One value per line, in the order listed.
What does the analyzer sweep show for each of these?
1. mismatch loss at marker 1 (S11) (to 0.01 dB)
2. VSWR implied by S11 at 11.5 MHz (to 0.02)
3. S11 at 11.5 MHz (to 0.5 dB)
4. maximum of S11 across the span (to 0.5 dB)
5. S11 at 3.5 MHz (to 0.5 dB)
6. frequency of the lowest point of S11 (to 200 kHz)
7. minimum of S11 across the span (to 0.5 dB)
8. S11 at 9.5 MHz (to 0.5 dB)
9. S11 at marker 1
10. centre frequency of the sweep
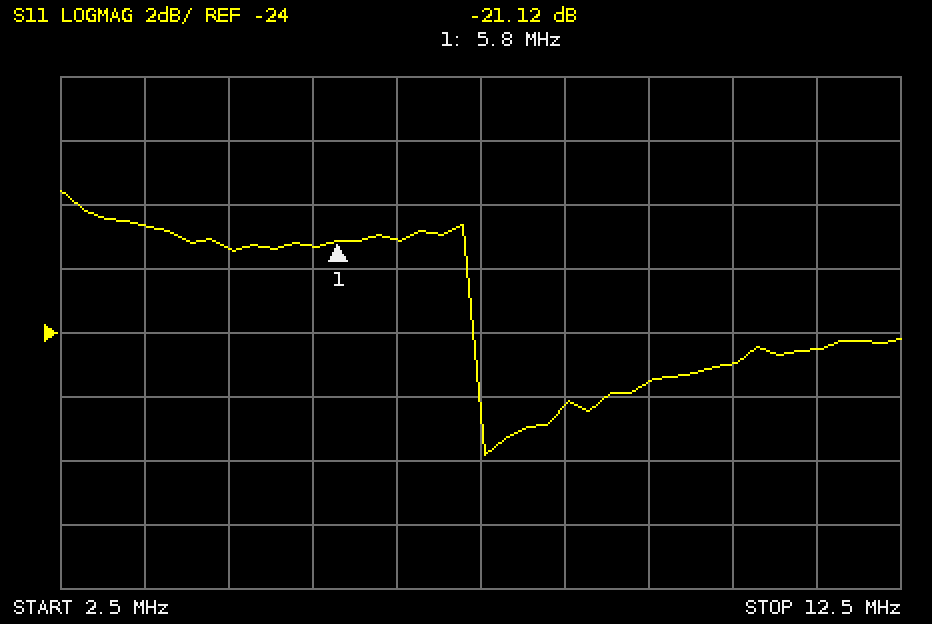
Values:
0.03 dB
1.12
-24.5 dB
-19.5 dB
-20.5 dB
7.6 MHz
-28.0 dB
-25.5 dB
-21.12 dB
7.5 MHz
